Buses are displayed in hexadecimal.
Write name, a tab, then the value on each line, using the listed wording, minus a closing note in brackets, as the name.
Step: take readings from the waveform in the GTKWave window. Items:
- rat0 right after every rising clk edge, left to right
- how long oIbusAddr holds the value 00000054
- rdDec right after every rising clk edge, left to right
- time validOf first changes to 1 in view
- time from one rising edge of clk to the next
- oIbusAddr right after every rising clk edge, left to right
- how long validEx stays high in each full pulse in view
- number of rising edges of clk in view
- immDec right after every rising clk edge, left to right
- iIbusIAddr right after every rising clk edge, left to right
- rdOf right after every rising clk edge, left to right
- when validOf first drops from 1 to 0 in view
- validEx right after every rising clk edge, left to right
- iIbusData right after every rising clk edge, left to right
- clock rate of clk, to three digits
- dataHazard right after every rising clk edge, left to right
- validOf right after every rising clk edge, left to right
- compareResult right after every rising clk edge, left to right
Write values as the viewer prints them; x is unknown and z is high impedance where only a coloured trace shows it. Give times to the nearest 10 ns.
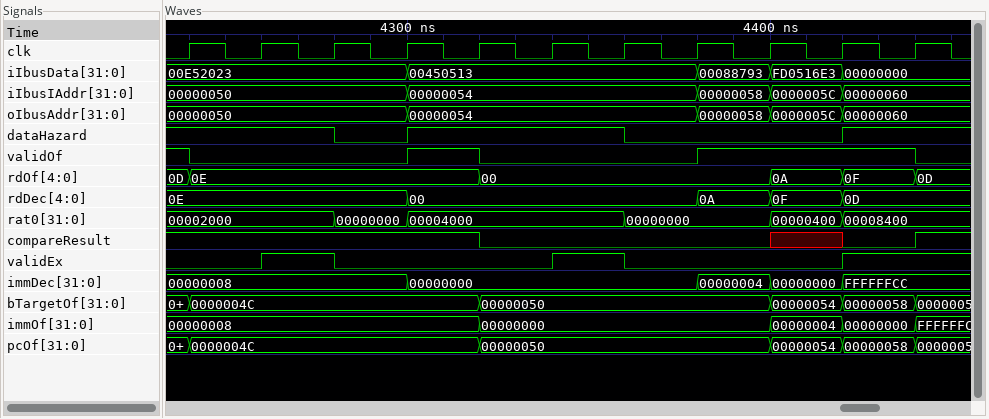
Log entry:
rat0 right after every rising clk edge, left to right	00002000, 00002000, 00000000, 00004000, 00004000, 00004000, 00000000, 00000000, 00000400, 00008400, 00008400
how long oIbusAddr holds the value 00000054	80 ns
rdDec right after every rising clk edge, left to right	0E, 0E, 0E, 00, 00, 00, 00, 0A, 0F, 0D, 0D
time validOf first changes to 1 in view	4300 ns
time from one rising edge of clk to the next	20 ns
oIbusAddr right after every rising clk edge, left to right	00000050, 00000050, 00000050, 00000054, 00000054, 00000054, 00000054, 00000058, 0000005C, 00000060, 00000060
how long validEx stays high in each full pulse in view	20 ns, 20 ns
number of rising edges of clk in view	11
immDec right after every rising clk edge, left to right	00000008, 00000008, 00000008, 00000000, 00000000, 00000000, 00000000, 00000004, 00000000, FFFFFFCC, FFFFFFCC
iIbusIAddr right after every rising clk edge, left to right	00000050, 00000050, 00000050, 00000054, 00000054, 00000054, 00000054, 00000058, 0000005C, 00000060, 00000060
rdOf right after every rising clk edge, left to right	0E, 0E, 0E, 0E, 00, 00, 00, 00, 0A, 0F, 0D
when validOf first drops from 1 to 0 in view	4240 ns
validEx right after every rising clk edge, left to right	0 1 0 0 0 1 0 0 0 1 1
iIbusData right after every rising clk edge, left to right	00E52023, 00E52023, 00E52023, 00450513, 00450513, 00450513, 00450513, 00088793, FD0516E3, 00000000, 00000000
clock rate of clk, to three digits	50.0 MHz
dataHazard right after every rising clk edge, left to right	1 1 0 1 1 1 0 0 0 1 1
validOf right after every rising clk edge, left to right	0 0 0 1 0 0 0 1 1 1 0
compareResult right after every rising clk edge, left to right	1 1 1 1 0 0 0 0 x 0 1
